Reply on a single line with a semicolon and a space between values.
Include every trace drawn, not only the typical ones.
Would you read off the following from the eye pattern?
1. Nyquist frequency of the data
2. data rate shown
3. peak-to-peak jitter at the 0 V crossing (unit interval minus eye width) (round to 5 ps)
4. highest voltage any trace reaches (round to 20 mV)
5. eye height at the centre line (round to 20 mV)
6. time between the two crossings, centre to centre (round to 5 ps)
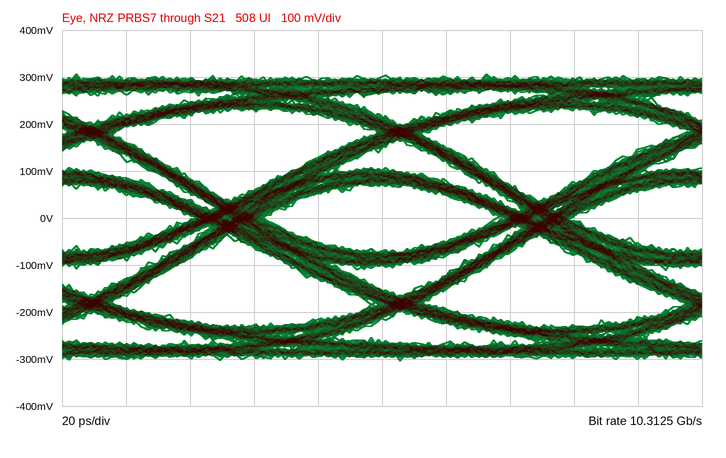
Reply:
5.15625 GHz; 10.3125 Gb/s; 25 ps; 300 mV; 140 mV; 95 ps
